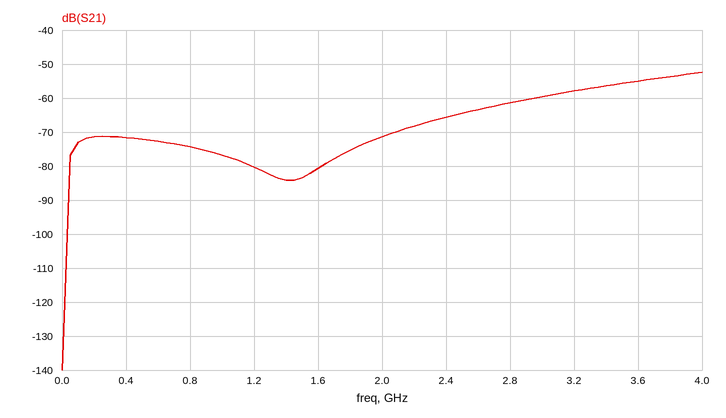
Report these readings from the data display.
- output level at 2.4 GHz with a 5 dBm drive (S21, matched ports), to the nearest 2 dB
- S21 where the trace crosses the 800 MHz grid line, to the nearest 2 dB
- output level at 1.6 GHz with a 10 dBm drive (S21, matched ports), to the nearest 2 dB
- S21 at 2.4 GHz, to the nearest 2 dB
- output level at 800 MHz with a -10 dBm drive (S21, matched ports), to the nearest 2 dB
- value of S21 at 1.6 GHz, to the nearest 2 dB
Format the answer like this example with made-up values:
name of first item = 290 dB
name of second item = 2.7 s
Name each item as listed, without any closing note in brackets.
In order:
output level at 2.4 GHz with a 5 dBm drive (S21, matched ports), to the nearest 2 dB = -60 dBm
S21 where the trace crosses the 800 MHz grid line, to the nearest 2 dB = -74 dB
output level at 1.6 GHz with a 10 dBm drive (S21, matched ports), to the nearest 2 dB = -70 dBm
S21 at 2.4 GHz, to the nearest 2 dB = -66 dB
output level at 800 MHz with a -10 dBm drive (S21, matched ports), to the nearest 2 dB = -84 dBm
value of S21 at 1.6 GHz, to the nearest 2 dB = -80 dB
